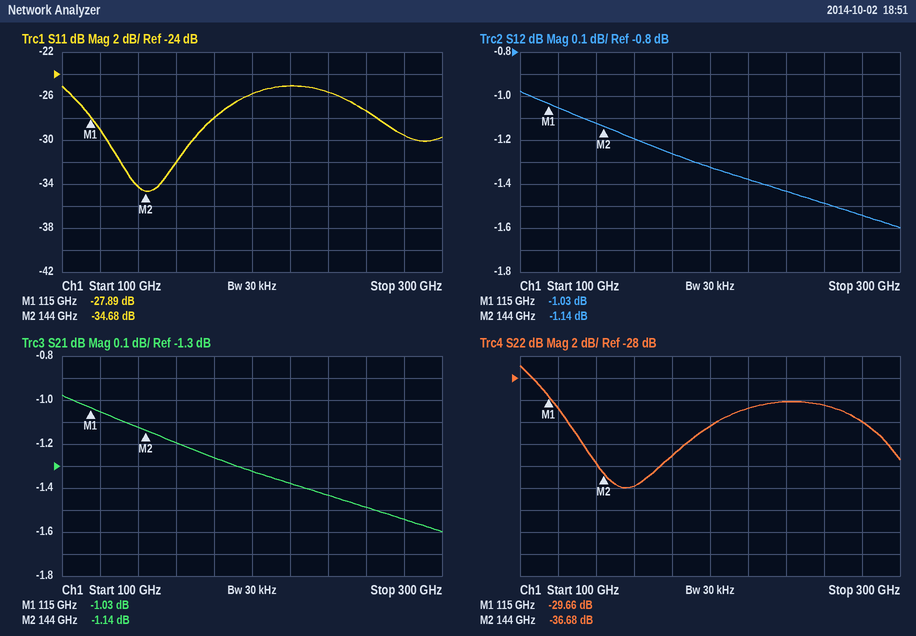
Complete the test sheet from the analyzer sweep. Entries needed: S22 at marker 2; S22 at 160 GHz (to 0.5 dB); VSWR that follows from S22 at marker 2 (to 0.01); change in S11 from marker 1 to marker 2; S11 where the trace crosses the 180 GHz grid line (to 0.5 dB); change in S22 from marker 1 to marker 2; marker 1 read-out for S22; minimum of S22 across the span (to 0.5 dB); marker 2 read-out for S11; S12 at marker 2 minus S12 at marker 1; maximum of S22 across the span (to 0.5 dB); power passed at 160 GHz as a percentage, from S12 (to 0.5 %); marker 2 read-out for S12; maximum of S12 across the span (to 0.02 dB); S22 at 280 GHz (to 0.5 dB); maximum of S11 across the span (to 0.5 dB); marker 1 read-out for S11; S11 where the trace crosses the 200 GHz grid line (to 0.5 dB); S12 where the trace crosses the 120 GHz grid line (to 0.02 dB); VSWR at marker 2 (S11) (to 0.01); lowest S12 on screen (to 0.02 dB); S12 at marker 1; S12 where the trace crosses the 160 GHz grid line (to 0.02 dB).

-36.68 dB
-38.0 dB
1.03
-6.79 dB
-28.0 dB
-7.02 dB
-29.66 dB
-38.0 dB
-34.68 dB
-0.11 dB
-27.0 dB
76.0 %
-1.14 dB
-0.98 dB
-32.0 dB
-25.0 dB
-27.89 dB
-26.0 dB
-1.06 dB
1.04
-1.60 dB
-1.03 dB
-1.20 dB
